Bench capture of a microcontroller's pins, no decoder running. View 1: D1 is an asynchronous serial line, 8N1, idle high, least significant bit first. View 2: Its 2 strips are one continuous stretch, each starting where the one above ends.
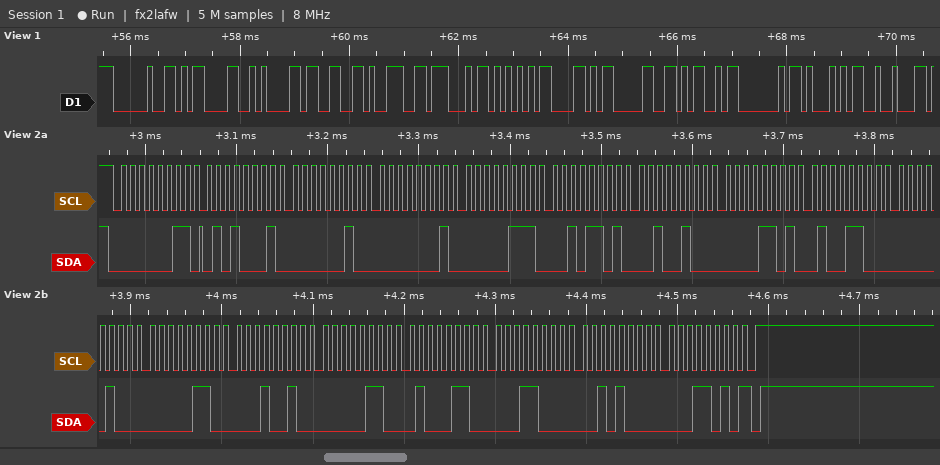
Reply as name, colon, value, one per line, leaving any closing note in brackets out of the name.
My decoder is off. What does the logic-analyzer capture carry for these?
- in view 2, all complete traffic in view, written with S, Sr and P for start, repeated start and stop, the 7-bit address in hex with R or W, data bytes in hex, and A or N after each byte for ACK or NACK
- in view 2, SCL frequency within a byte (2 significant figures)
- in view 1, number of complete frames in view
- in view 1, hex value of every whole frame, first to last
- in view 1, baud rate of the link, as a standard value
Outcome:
in view 2, all complete traffic in view, written with S, Sr and P for start, repeated start and stop, the 7-bit address in hex with R or W, data bytes in hex, and A or N after each byte for ACK or NACK: S 01R A 51 A 02 A 01 A 07 A 2D A 24 A 0D A 4C A 04 A 06 A 12 A 06 A 46 A 18 A 28 A 1A N P
in view 2, SCL frequency within a byte: 100 kHz
in view 1, number of complete frames in view: 13
in view 1, hex value of every whole frame, first to last: 20 0D 0A 33 39 47 55 58 30 4D 40 51 12
in view 1, baud rate of the link, as a standard value: 9600 baud
